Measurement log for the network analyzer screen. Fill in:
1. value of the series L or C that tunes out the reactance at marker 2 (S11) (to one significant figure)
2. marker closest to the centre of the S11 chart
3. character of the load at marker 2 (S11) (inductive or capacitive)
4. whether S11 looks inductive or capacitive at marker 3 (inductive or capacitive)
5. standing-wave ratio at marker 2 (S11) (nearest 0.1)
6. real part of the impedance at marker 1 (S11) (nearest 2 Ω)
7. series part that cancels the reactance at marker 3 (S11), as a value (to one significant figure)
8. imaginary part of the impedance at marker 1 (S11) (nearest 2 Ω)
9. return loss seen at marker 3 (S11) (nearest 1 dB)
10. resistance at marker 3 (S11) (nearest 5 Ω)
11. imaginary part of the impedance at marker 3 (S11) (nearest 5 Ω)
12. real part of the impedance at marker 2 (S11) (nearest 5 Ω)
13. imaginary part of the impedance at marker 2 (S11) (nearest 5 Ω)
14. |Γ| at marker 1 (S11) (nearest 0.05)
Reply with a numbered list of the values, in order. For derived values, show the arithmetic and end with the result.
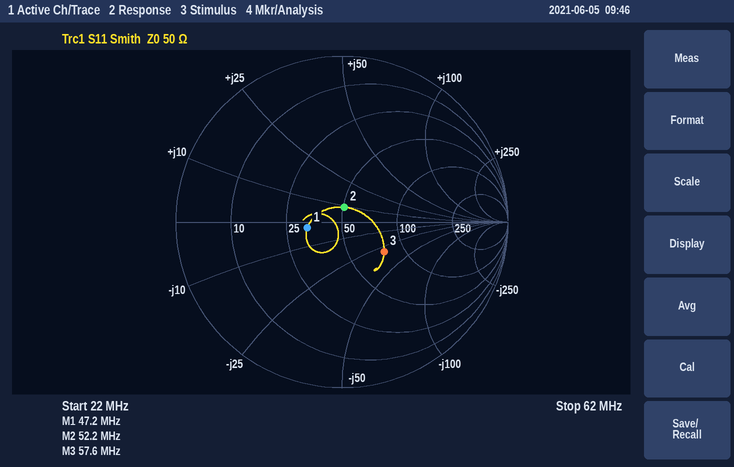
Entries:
1. C = 1/(2π × 52.2 MHz × 10 Ω) ≈ 305 pF, so 300 pF to one significant figure
2. marker 2
3. inductive
4. capacitive
5. 1.2
6. 32 Ω
7. L = 30 Ω/(2π × 57.6 MHz) ≈ 82.9 nH, so 80 nH to one significant figure
8. -2 Ω
9. 10 dB
10. 75 Ω
11. -30 Ω
12. 50 Ω
13. +10 Ω
14. 0.20
